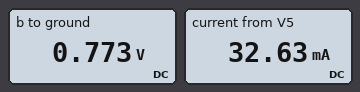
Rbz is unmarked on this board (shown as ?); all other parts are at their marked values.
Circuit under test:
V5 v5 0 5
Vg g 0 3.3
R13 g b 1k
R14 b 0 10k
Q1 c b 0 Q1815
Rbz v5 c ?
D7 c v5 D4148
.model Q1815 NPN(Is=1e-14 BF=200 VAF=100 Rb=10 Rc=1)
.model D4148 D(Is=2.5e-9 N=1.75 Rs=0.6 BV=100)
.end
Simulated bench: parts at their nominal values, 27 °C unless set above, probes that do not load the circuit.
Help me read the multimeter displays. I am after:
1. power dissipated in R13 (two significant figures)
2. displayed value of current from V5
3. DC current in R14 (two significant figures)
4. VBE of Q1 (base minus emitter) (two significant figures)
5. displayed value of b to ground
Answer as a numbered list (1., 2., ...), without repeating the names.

1. 6.4 mW
2. 32.63 mA
3. 77 µA
4. 770 mV
5. 0.773 V
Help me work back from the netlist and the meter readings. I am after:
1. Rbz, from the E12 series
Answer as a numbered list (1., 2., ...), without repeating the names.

1. 150 Ω
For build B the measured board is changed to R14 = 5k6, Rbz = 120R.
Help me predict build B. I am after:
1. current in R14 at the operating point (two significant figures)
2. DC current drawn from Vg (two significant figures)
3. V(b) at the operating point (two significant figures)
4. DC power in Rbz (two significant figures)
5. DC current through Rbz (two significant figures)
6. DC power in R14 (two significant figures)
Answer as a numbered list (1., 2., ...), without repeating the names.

1. 140 µA
2. 2.5 mA
3. 780 mV
4. 200 mW
5. 41 mA
6. 110 µW
